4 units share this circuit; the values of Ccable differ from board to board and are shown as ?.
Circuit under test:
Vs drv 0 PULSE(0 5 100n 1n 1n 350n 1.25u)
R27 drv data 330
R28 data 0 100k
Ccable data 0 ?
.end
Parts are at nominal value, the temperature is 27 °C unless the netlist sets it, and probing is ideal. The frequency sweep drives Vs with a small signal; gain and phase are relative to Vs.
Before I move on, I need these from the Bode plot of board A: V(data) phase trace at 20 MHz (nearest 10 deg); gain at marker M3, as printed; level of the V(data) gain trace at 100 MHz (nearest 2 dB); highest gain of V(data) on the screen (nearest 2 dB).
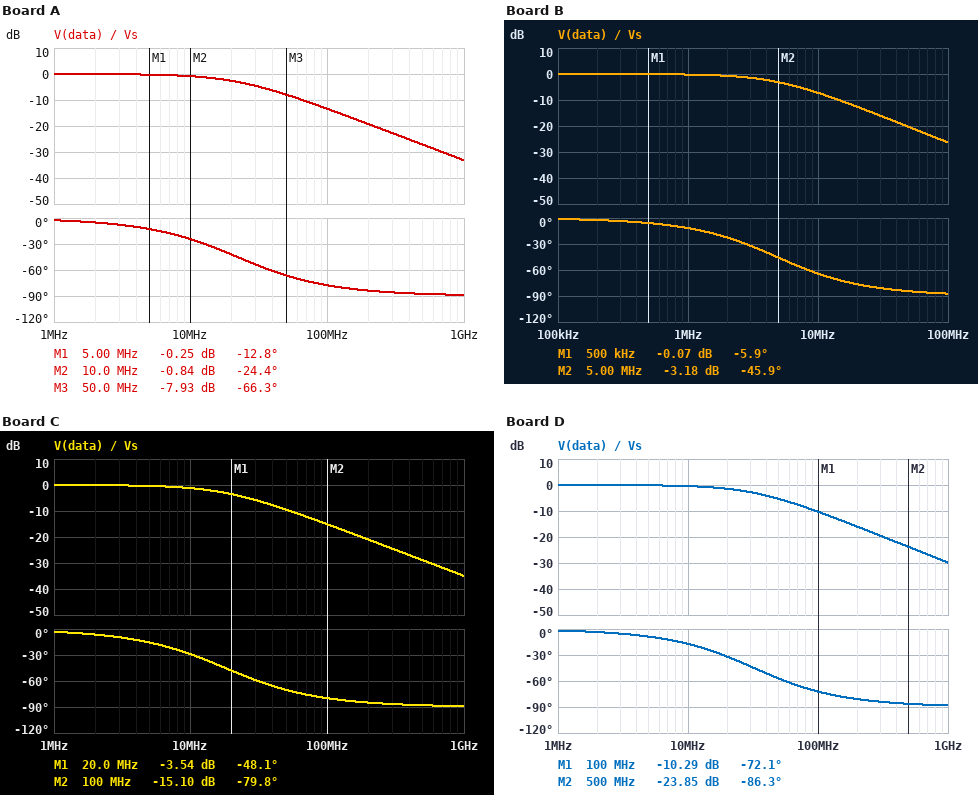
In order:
-40 deg
-7.93 dB
-14 dB
0 dB
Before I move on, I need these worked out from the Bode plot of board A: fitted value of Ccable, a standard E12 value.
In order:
22 pF
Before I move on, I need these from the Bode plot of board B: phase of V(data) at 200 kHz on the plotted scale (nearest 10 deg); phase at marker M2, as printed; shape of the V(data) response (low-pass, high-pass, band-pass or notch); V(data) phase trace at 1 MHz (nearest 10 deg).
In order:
0 deg
-45.9 deg
low-pass
-10 deg
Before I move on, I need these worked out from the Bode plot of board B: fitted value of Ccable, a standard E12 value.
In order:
100 pF
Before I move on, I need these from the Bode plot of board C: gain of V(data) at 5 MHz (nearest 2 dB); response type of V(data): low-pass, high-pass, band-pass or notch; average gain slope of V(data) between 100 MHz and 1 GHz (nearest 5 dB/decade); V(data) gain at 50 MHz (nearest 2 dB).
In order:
0 dB
low-pass
-20 dB/decade
-10 dB
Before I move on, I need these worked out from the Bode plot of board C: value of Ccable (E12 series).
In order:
27 pF
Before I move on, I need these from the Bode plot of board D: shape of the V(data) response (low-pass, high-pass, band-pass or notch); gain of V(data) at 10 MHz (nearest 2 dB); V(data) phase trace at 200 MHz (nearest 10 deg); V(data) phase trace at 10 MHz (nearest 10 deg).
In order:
low-pass
0 dB
-80 deg
-20 deg
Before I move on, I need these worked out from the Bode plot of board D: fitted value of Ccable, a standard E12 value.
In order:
15 pF
